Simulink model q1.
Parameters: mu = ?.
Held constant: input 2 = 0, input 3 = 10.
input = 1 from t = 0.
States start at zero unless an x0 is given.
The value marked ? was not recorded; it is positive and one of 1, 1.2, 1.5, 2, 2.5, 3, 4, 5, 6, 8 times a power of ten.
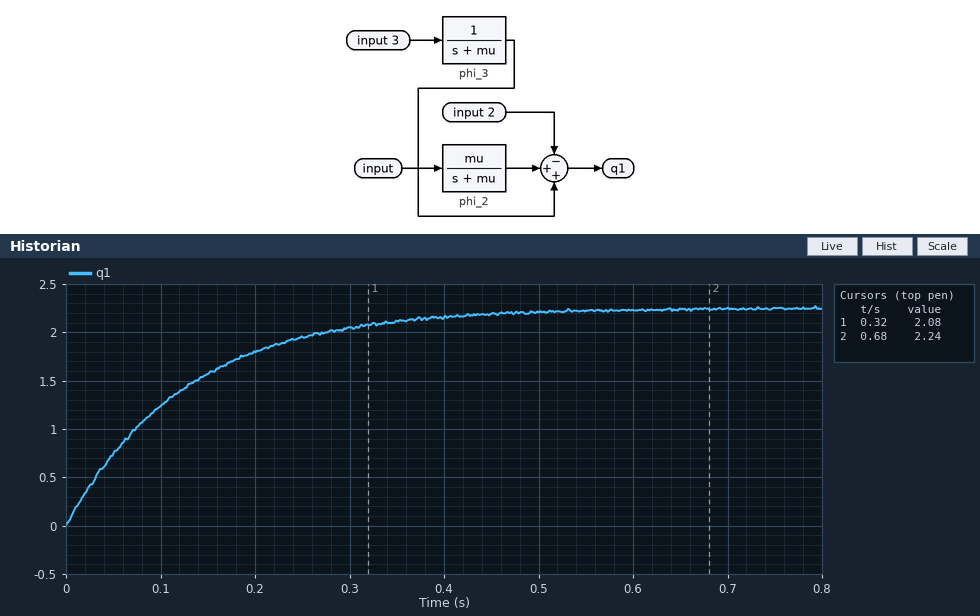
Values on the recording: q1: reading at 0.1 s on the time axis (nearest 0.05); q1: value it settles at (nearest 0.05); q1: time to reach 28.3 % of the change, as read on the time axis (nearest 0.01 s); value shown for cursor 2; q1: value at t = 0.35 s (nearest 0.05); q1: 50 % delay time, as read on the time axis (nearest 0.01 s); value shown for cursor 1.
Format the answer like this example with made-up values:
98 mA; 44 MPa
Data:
1.25; 2.25; 0.04 s; 2.24; 2.10; 0.09 s; 2.08
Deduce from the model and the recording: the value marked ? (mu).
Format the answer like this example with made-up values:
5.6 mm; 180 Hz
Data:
8
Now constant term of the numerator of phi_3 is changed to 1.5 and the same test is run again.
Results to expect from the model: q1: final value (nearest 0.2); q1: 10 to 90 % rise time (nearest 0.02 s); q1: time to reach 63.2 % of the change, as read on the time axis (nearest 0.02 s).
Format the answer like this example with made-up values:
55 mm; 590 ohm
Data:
2.8; 0.28 s; 0.12 s
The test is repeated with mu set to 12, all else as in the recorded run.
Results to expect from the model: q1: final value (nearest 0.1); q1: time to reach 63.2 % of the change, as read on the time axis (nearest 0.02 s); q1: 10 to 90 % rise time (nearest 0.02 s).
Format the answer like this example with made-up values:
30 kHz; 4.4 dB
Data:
1.8; 0.08 s; 0.18 s
